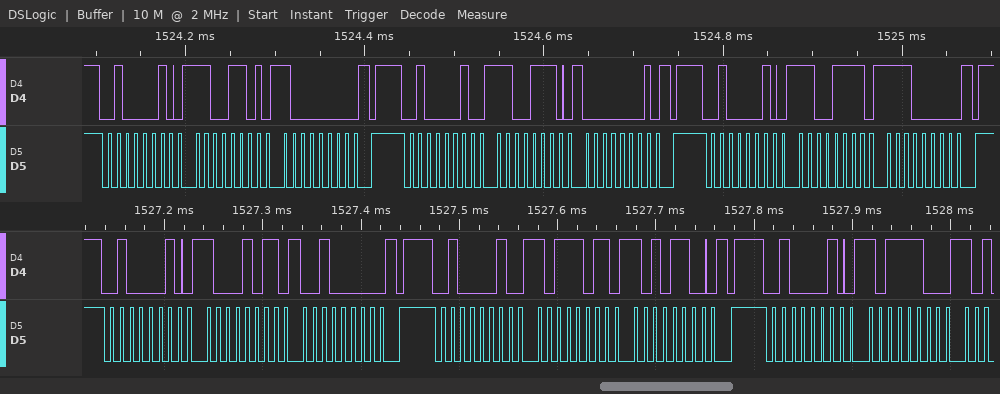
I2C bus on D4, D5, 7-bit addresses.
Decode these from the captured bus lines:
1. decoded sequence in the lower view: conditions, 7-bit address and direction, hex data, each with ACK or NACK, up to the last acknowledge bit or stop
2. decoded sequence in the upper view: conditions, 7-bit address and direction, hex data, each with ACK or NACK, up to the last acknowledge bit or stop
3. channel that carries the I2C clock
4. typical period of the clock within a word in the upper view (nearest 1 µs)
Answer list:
start, address 21 write ACK, 8B ACK, 20 ACK, stop, start, address 21 write ACK, BB ACK, AC ACK, stop, start, address 21 write ACK, BC ACK
start, address 21 write ACK, CD ACK, 80 ACK, stop, start, address 21 write ACK, CE ACK, 01 ACK, stop, start, address 21 write ACK, CF ACK, E0 ACK, stop
D5
10 µs
